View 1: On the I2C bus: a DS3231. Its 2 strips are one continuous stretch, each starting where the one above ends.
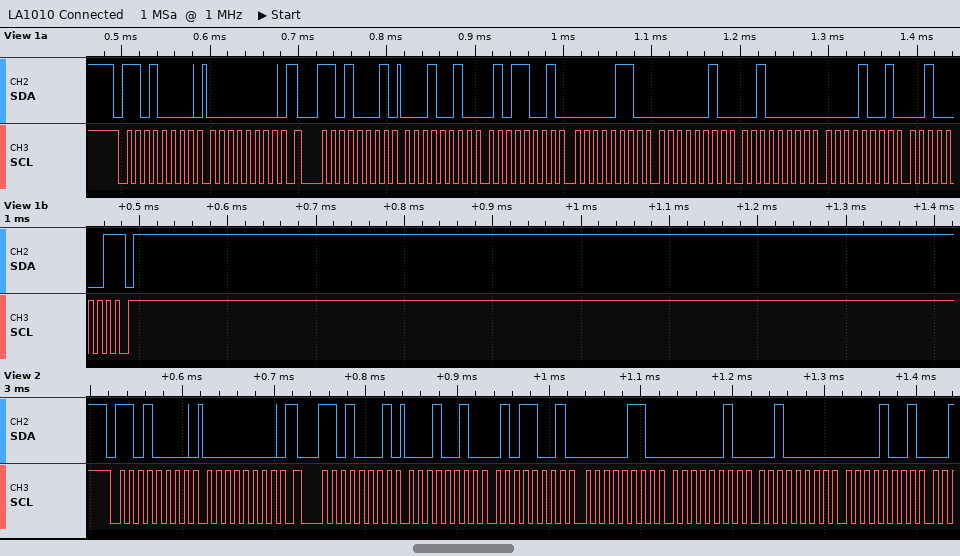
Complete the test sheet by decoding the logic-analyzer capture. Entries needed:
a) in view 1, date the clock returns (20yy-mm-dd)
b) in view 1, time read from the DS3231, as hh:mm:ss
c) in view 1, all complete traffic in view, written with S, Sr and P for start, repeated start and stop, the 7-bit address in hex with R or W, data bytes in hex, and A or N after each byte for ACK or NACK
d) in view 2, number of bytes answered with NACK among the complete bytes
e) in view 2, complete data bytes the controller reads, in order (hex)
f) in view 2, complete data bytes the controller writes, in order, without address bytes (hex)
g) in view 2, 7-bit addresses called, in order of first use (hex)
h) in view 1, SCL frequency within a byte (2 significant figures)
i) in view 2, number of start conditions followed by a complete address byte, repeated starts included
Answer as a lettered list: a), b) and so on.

a) 2021-09-20
b) 06:59:12
c) S 68W A 00 A Sr 68R A 12 A 59 A 06 A 02 A 20 A 09 A 21 N P
d) 0
e) 12 59 06 02 20 09
f) 00
g) 0x68
h) 100 kHz
i) 2
